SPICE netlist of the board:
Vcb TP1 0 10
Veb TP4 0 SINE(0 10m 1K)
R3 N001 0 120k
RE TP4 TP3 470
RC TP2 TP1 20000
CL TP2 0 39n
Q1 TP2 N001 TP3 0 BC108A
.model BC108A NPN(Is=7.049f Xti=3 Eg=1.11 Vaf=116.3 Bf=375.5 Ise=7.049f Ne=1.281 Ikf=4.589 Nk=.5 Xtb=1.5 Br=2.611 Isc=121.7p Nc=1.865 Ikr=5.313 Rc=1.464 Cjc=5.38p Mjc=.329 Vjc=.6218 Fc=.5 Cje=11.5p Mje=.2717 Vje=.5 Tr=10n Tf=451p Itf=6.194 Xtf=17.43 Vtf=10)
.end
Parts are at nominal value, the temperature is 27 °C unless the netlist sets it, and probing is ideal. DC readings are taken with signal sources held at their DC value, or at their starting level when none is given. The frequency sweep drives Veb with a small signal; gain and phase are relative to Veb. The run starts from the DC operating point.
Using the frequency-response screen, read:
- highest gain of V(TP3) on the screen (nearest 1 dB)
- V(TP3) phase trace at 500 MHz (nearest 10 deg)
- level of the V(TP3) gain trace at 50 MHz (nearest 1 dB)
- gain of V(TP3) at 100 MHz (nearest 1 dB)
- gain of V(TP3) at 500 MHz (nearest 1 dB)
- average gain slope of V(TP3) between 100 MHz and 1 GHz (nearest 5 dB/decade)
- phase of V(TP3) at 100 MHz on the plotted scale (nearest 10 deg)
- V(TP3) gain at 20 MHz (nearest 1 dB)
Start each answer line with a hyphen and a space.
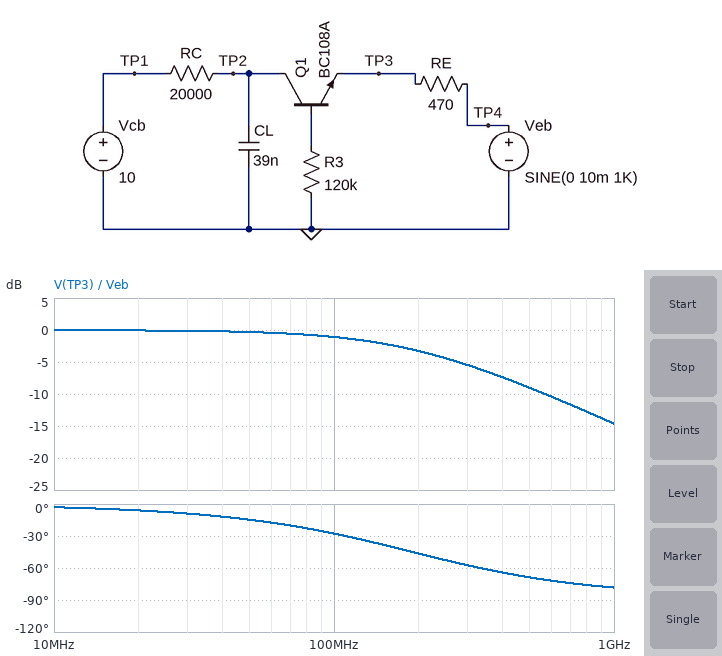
- 0 dB
- -70 deg
- 0 dB
- -1 dB
- -9 dB
- -15 dB/decade
- -30 deg
- 0 dB
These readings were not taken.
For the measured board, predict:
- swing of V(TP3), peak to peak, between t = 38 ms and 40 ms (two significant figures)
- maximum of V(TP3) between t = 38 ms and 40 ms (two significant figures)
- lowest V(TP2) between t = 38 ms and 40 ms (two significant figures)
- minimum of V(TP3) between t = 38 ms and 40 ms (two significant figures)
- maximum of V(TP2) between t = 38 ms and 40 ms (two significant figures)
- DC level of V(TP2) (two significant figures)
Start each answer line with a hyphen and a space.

- 20 mV
- 10 mV
- 10 V
- -10 mV
- 10 V
- 10 V
